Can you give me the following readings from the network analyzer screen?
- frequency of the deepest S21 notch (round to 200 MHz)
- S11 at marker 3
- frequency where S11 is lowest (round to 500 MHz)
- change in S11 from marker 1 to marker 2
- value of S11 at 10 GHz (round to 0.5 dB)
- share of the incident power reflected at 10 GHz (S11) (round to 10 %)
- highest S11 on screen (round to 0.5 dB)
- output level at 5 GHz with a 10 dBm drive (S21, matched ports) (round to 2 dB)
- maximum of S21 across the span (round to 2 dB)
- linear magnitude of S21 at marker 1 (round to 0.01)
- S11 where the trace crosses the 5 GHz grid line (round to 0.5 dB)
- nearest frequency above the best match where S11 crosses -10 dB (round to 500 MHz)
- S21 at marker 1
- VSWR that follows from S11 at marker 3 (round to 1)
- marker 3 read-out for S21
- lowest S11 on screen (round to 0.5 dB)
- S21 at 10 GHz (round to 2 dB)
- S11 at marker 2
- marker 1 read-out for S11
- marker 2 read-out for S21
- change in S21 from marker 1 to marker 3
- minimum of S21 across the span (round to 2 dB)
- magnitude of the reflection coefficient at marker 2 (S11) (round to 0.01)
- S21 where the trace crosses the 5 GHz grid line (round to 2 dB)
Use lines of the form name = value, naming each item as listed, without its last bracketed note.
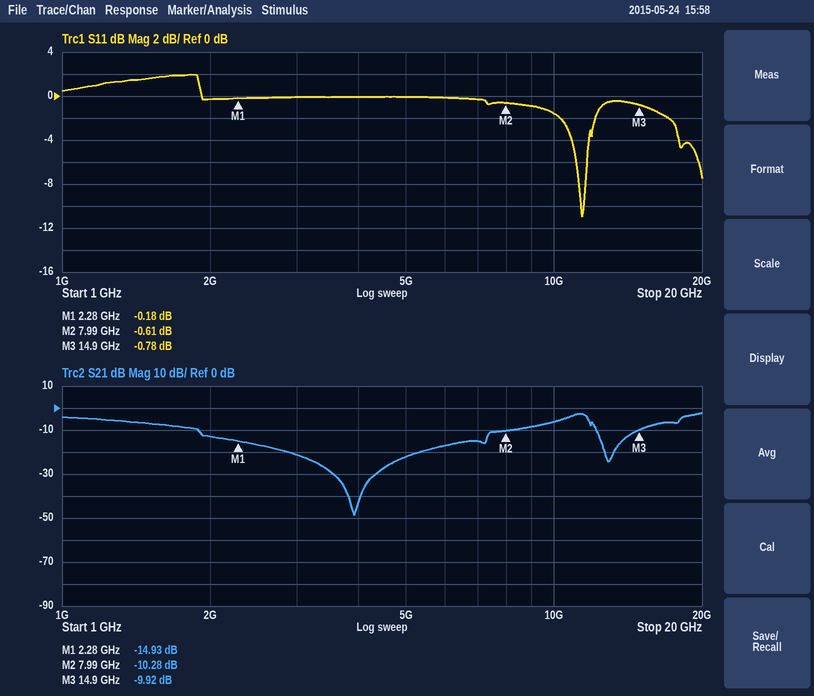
frequency of the deepest S21 notch = 4.0 GHz
S11 at marker 3 = -0.78 dB
frequency where S11 is lowest = 11.5 GHz
change in S11 from marker 1 to marker 2 = -0.43 dB
value of S11 at 10 GHz = -1.5 dB
share of the incident power reflected at 10 GHz (S11) = 70 %
highest S11 on screen = 2.0 dB
output level at 5 GHz with a 10 dBm drive (S21, matched ports) = -12 dBm
maximum of S21 across the span = -2 dB
linear magnitude of S21 at marker 1 = 0.18
S11 where the trace crosses the 5 GHz grid line = 0.0 dB
nearest frequency above the best match where S11 crosses -10 dB = 11.5 GHz
S21 at marker 1 = -14.93 dB
VSWR that follows from S11 at marker 3 = 22
marker 3 read-out for S21 = -9.92 dB
lowest S11 on screen = -11.0 dB
S21 at 10 GHz = -6 dB
S11 at marker 2 = -0.61 dB
marker 1 read-out for S11 = -0.18 dB
marker 2 read-out for S21 = -10.28 dB
change in S21 from marker 1 to marker 3 = 5.01 dB
minimum of S21 across the span = -48 dB
magnitude of the reflection coefficient at marker 2 (S11) = 0.93
S21 where the trace crosses the 5 GHz grid line = -22 dB
